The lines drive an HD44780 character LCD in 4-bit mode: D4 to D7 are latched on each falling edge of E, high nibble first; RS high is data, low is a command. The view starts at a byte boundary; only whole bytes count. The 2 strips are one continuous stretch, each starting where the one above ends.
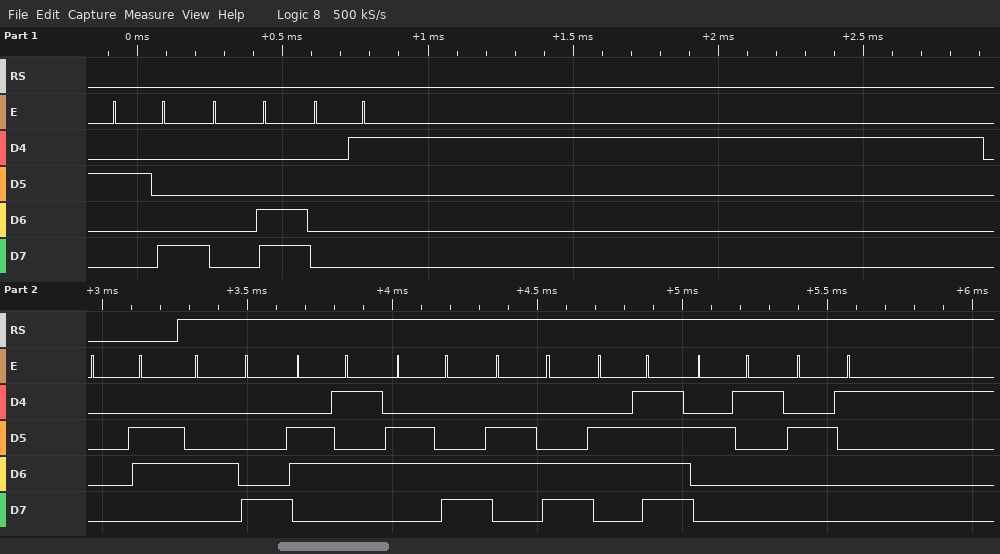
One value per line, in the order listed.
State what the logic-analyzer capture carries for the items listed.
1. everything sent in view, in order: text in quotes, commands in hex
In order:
0x28 0x0C 0x01 0x06 "Hello!!"
